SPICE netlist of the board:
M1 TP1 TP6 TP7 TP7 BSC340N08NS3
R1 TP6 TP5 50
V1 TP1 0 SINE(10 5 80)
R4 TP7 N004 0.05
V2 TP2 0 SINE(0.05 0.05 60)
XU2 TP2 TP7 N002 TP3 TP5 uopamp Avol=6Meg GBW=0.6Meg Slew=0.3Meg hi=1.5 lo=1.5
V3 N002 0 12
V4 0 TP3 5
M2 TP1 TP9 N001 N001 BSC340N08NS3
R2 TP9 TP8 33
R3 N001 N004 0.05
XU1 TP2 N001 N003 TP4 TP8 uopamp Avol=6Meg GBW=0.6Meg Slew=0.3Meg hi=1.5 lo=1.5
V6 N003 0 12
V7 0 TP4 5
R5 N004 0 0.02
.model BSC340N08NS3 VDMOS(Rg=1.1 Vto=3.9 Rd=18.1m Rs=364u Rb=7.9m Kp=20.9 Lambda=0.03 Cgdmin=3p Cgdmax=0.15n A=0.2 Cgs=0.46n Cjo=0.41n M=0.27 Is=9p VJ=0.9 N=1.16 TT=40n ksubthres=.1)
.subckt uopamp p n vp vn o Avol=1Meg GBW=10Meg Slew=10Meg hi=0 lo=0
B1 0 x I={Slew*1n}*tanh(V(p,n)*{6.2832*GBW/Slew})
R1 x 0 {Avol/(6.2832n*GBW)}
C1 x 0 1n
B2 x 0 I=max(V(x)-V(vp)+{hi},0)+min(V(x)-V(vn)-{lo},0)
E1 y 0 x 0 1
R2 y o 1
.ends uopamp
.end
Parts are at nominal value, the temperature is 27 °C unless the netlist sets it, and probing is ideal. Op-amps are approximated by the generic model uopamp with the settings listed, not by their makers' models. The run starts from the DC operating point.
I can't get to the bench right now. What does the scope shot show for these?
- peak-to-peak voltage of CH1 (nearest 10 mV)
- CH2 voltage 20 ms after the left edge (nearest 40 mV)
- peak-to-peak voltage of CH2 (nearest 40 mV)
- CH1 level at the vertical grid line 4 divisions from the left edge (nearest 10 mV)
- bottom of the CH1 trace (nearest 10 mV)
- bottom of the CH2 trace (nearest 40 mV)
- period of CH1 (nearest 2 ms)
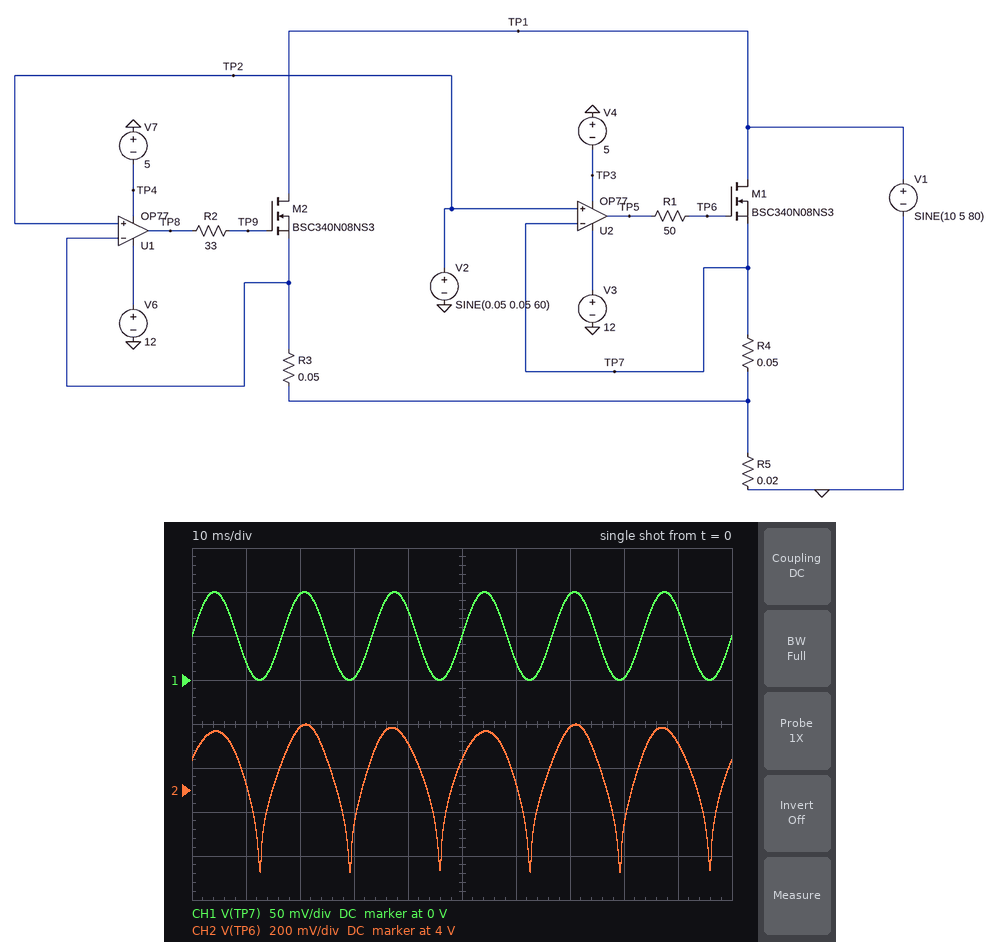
100 mV
4.28 V
680 mV
80 mV
0 V
3.64 V
16 ms
